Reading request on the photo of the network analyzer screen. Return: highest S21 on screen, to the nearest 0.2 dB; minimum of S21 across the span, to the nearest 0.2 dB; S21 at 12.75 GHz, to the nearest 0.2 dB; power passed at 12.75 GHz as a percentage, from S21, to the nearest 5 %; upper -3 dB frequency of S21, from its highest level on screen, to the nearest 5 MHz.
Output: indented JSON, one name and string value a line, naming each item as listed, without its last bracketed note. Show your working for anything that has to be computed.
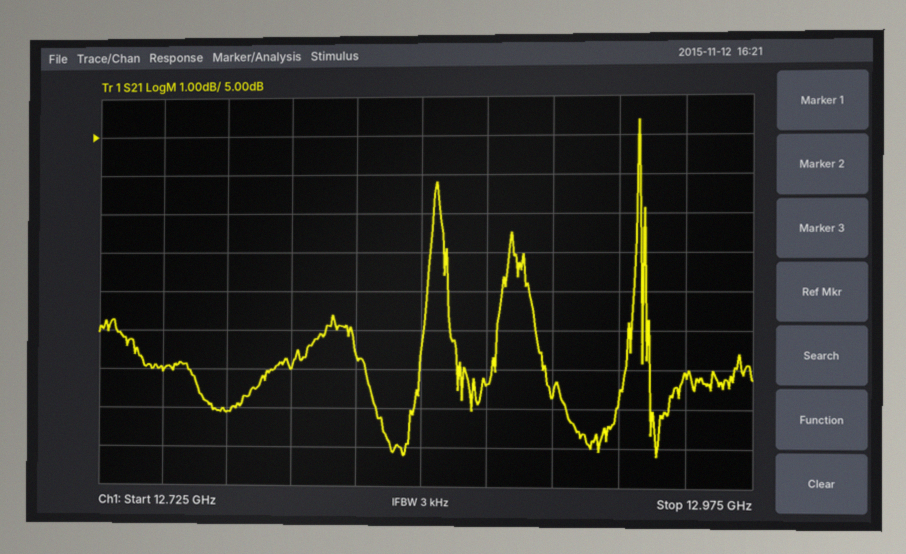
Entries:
{
  "highest S21 on screen, to the nearest 0.2 dB": "5.4 dB",
  "minimum of S21 across the span, to the nearest 0.2 dB": "-3.2 dB",
  "S21 at 12.75 GHz, to the nearest 0.2 dB": "-1.0 dB",
  "power passed at 12.75 GHz as a percentage, from S21, to the nearest 5 %": "10^(-1/10) ≈ 79.4 %, so 80 % to the nearest 5 %",
  "upper -3 dB frequency of S21, from its highest level on screen, to the nearest 5 MHz": "12.935 GHz"
}
